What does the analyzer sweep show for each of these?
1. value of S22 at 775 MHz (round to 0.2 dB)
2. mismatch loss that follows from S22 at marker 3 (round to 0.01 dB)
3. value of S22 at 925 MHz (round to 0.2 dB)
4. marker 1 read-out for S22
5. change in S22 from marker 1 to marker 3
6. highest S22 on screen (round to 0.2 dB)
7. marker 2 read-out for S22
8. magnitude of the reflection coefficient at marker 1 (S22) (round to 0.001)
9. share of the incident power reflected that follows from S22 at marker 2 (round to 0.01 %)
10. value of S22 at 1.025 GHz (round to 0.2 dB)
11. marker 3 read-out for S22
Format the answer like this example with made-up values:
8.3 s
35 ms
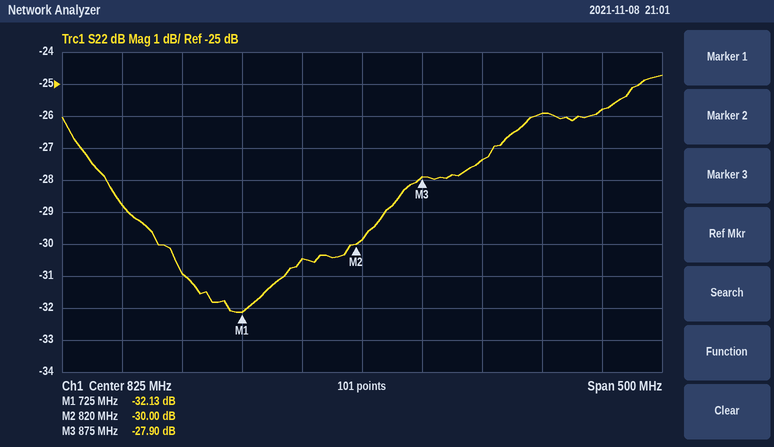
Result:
-30.4 dB
0.01 dB
-27.4 dB
-32.13 dB
4.23 dB
-24.8 dB
-30.00 dB
0.025
0.10 %
-25.8 dB
-27.90 dB
